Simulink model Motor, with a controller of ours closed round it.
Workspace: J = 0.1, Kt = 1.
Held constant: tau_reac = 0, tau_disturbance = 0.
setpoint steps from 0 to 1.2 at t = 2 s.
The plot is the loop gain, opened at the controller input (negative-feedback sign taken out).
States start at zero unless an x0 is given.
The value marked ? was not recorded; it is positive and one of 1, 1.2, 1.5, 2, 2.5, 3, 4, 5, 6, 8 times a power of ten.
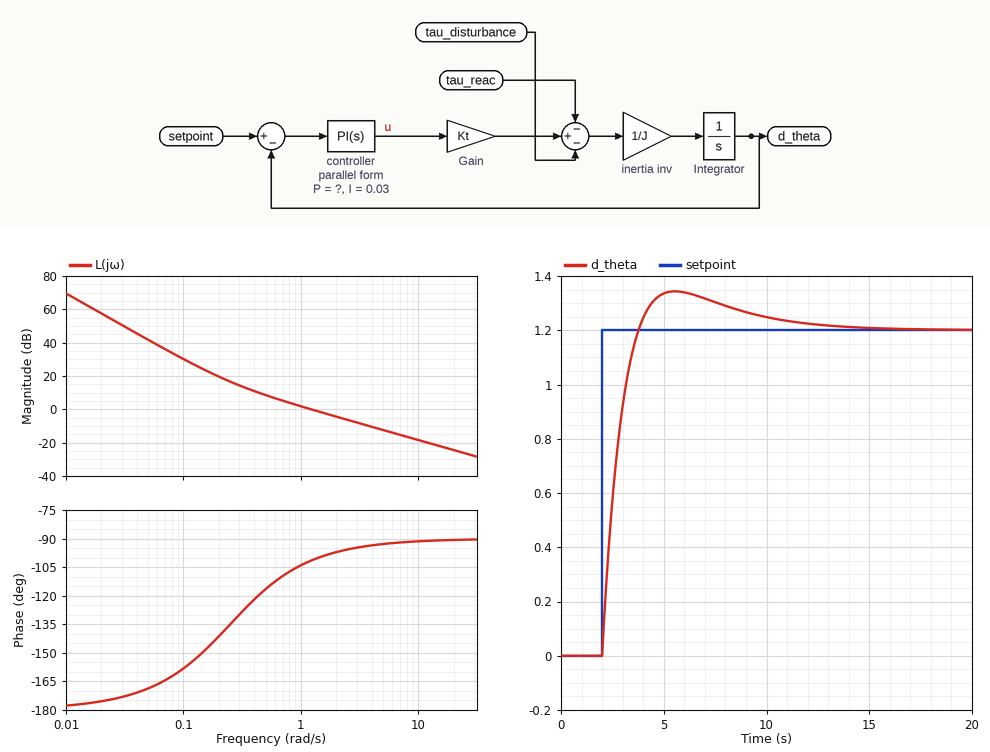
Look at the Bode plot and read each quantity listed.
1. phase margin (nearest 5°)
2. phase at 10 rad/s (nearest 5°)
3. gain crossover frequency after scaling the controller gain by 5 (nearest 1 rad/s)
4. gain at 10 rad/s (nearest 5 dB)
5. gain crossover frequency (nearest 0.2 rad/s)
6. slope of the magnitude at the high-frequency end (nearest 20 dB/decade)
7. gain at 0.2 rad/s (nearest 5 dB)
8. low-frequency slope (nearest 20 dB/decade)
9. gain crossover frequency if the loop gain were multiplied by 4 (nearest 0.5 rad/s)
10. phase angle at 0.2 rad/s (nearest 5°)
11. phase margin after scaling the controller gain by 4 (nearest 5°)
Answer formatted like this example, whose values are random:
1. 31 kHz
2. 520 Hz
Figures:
1. 80°
2. -90°
3. 6 rad/s
4. -20 dB
5. 1.2 rad/s
6. -20 dB/decade
7. 20 dB
8. -40 dB/decade
9. 5.0 rad/s
10. -140°
11. 85°
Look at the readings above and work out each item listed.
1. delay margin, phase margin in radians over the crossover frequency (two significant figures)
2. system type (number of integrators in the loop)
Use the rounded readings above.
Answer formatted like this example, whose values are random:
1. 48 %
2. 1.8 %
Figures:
1. 1.2 s
2. 2
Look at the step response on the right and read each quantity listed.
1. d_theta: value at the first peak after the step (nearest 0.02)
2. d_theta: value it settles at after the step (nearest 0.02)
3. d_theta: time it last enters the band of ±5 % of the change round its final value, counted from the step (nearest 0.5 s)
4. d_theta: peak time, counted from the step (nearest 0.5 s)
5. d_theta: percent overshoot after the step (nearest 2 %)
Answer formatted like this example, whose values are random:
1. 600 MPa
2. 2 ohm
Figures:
1. 1.34
2. 1.20
3. 7.5 s
4. 3.5 s
5. 12 %
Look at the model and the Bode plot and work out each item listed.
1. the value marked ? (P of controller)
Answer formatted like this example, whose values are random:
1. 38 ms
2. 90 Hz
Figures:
1. 0.12
